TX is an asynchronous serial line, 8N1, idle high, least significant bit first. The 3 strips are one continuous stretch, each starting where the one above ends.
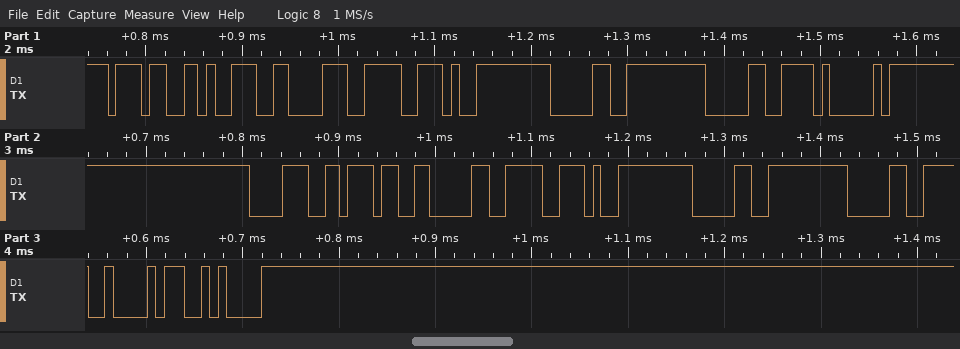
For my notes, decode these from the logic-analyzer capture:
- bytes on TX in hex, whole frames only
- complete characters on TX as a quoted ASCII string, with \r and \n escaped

37 39 38 2E 30 30 41 38 37 30 2E 30 30 42 0A
"798.00A870.00B\n"
